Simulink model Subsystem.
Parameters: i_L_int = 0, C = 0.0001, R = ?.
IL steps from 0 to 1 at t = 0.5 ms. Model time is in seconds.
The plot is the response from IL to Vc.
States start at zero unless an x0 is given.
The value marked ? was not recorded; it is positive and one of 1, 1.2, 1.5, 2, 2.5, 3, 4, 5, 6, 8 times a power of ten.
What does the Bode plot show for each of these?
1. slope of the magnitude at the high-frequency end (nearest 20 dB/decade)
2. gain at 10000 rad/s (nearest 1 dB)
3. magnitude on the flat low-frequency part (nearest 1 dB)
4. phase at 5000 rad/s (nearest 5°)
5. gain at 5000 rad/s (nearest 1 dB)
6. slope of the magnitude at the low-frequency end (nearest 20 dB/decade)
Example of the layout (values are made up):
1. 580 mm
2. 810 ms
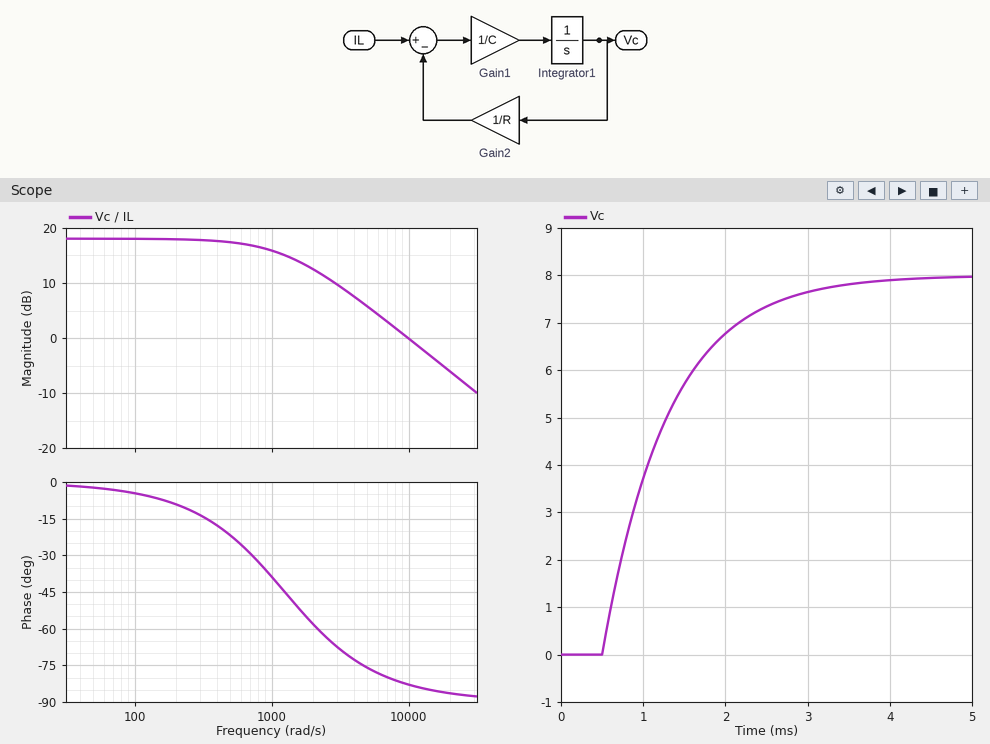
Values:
1. -20 dB/decade
2. 0 dB
3. 18 dB
4. -75°
5. 6 dB
6. 0 dB/decade
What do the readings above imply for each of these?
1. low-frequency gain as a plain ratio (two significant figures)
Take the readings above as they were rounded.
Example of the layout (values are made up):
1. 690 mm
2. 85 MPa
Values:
1. 7.9
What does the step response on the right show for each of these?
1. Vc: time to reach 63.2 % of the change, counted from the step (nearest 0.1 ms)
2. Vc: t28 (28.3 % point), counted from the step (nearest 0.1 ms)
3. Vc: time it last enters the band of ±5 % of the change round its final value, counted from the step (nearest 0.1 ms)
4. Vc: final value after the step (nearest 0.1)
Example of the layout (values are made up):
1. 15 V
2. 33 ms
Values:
1. 0.8 ms
2. 0.3 ms
3. 2.4 ms
4. 8.0
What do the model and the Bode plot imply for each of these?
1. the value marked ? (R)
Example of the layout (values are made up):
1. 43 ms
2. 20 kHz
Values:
1. 8
